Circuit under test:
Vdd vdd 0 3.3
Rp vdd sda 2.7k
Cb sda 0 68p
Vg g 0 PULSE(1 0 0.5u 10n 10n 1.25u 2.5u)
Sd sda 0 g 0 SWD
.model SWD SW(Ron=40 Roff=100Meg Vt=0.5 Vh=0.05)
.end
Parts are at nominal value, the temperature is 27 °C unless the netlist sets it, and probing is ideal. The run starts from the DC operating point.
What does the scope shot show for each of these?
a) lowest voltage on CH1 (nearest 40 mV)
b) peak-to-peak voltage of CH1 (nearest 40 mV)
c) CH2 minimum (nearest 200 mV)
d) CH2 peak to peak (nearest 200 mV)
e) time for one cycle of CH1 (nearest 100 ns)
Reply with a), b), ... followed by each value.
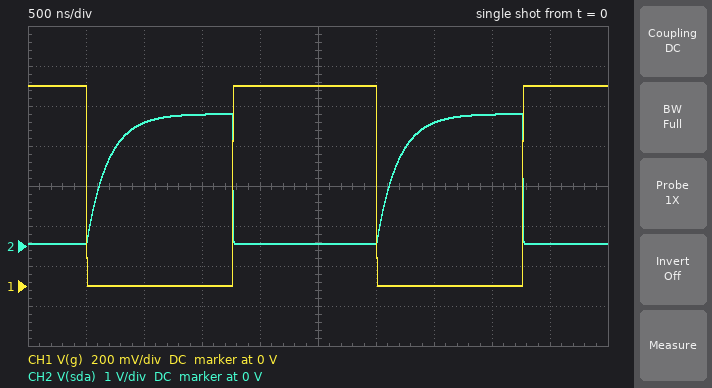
a) 0 V
b) 1.00 V
c) 0 V
d) 3.2 V
e) 2.5 µs
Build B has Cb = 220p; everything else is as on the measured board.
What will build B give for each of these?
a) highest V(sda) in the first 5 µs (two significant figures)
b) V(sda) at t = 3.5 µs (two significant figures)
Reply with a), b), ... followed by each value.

a) 2.9 V
b) 1.9 V
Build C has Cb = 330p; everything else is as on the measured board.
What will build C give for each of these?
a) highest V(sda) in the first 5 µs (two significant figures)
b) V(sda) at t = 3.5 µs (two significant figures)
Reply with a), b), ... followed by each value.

a) 2.5 V
b) 1.4 V
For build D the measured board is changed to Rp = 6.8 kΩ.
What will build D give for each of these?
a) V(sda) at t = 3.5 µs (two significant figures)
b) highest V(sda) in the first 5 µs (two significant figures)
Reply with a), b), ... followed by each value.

a) 2.2 V
b) 3.1 V
